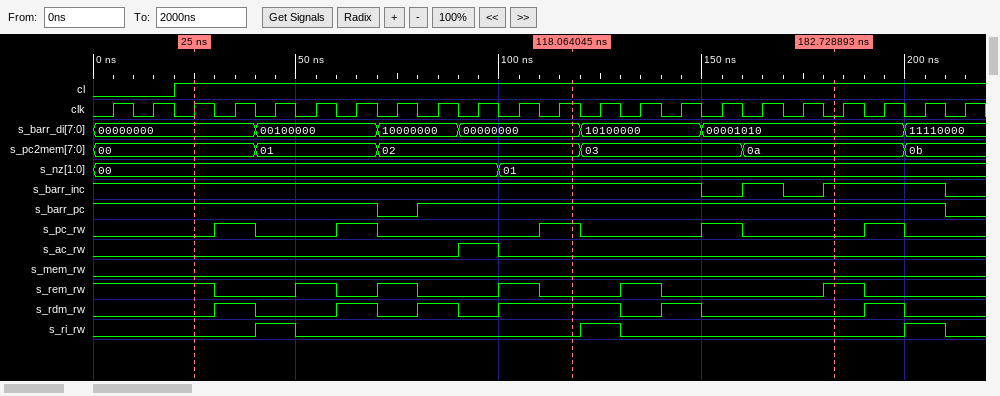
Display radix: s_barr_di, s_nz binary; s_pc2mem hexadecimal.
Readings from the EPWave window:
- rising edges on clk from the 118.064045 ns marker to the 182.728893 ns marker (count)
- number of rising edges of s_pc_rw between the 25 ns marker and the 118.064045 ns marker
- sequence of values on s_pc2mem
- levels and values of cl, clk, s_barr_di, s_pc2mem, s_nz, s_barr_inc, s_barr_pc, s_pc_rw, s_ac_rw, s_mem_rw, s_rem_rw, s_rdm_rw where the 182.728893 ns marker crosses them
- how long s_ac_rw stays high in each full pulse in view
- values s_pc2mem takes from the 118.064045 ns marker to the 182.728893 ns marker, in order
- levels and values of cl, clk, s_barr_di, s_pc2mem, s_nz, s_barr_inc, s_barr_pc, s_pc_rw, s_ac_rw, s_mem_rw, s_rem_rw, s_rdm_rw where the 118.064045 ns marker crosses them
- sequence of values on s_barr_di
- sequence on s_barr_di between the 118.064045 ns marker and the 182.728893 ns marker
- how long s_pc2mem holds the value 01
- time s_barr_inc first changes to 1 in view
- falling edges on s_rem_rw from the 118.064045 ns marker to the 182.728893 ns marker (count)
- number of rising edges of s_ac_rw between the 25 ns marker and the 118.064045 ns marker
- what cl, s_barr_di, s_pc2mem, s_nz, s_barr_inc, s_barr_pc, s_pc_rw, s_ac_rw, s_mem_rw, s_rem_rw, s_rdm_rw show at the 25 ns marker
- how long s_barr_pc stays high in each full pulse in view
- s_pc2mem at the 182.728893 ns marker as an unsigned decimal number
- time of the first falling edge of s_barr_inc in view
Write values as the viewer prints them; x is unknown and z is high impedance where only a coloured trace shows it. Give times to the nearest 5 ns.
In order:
6
3
00, 01, 02, 03, 0a, 0b
cl=1, clk=0, s_barr_di=00001010, s_pc2mem=0a, s_nz=01, s_barr_inc=1, s_barr_pc=1, s_pc_rw=0, s_ac_rw=0, s_mem_rw=0, s_rem_rw=1, s_rdm_rw=0
10 ns
02, 03, 0a
cl=1, clk=1, s_barr_di=00000000, s_pc2mem=02, s_nz=01, s_barr_inc=1, s_barr_pc=1, s_pc_rw=1, s_ac_rw=0, s_mem_rw=0, s_rem_rw=0, s_rdm_rw=1
00000000, 00100000, 10000000, 00000000, 10100000, 00001010, 11110000
00000000, 10100000, 00001010
30 ns
160 ns
1
1
cl=1, s_barr_di=00000000, s_pc2mem=00, s_nz=00, s_barr_inc=1, s_barr_pc=1, s_pc_rw=0, s_ac_rw=0, s_mem_rw=0, s_rem_rw=1, s_rdm_rw=0
130 ns
10
150 ns
